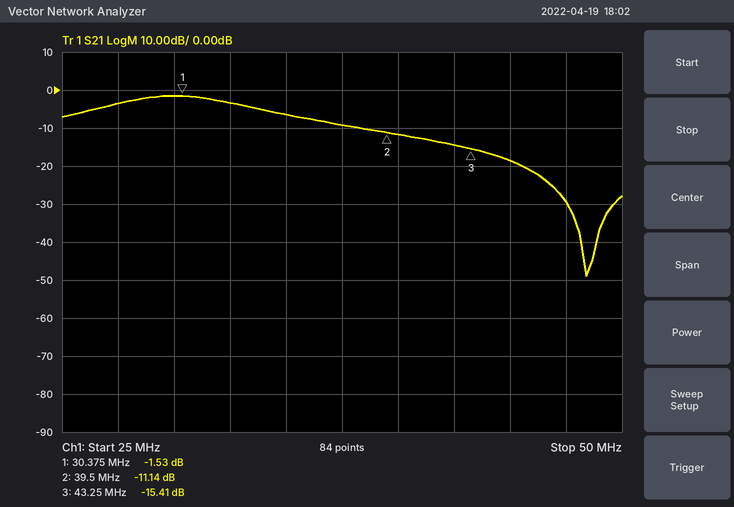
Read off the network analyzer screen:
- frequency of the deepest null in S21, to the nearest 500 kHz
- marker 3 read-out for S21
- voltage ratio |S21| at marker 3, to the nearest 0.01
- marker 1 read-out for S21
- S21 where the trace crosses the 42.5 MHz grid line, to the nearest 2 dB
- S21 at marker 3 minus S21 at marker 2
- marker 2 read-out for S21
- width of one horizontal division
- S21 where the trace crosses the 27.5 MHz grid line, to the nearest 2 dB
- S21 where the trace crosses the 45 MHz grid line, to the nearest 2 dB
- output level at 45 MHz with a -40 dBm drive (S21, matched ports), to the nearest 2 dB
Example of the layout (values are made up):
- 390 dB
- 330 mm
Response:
- 48.5 MHz
- -15.41 dB
- 0.17
- -1.53 dB
- -14 dB
- -4.27 dB
- -11.14 dB
- 2.5 MHz
- -4 dB
- -18 dB
- -58 dBm
